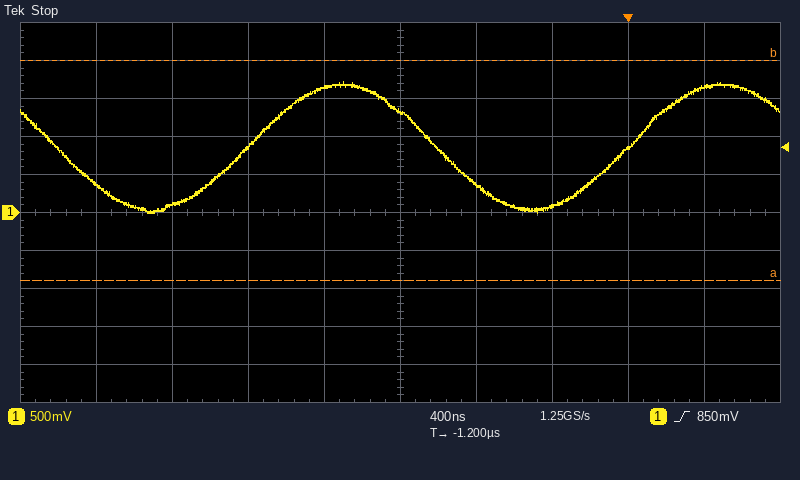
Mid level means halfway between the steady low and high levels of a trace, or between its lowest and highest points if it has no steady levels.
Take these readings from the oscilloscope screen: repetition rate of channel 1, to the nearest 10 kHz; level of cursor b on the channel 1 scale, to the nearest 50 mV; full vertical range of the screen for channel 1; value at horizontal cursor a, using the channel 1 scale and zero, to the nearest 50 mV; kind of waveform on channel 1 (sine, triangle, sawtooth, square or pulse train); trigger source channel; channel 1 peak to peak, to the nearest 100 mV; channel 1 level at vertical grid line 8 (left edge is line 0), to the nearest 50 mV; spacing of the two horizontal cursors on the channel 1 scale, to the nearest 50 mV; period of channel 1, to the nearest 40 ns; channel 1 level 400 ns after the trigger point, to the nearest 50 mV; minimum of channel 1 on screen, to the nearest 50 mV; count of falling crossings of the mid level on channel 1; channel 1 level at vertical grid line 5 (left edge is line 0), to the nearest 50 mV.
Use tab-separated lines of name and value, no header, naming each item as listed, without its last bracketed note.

repetition rate of channel 1, to the nearest 10 kHz	500 kHz
level of cursor b on the channel 1 scale, to the nearest 50 mV	2.00 V
full vertical range of the screen for channel 1	5 V
value at horizontal cursor a, using the channel 1 scale and zero, to the nearest 50 mV	-900 mV
kind of waveform on channel 1	sine
trigger source channel	channel 1
channel 1 peak to peak, to the nearest 100 mV	1.70 V
channel 1 level at vertical grid line 8 (left edge is line 0), to the nearest 50 mV	850 mV
spacing of the two horizontal cursors on the channel 1 scale, to the nearest 50 mV	2.90 V
period of channel 1, to the nearest 40 ns	2.00 µs
channel 1 level 400 ns after the trigger point, to the nearest 50 mV	1.65 V
minimum of channel 1 on screen, to the nearest 50 mV	0 mV
count of falling crossings of the mid level on channel 1	2
channel 1 level at vertical grid line 5 (left edge is line 0), to the nearest 50 mV	1.35 V
